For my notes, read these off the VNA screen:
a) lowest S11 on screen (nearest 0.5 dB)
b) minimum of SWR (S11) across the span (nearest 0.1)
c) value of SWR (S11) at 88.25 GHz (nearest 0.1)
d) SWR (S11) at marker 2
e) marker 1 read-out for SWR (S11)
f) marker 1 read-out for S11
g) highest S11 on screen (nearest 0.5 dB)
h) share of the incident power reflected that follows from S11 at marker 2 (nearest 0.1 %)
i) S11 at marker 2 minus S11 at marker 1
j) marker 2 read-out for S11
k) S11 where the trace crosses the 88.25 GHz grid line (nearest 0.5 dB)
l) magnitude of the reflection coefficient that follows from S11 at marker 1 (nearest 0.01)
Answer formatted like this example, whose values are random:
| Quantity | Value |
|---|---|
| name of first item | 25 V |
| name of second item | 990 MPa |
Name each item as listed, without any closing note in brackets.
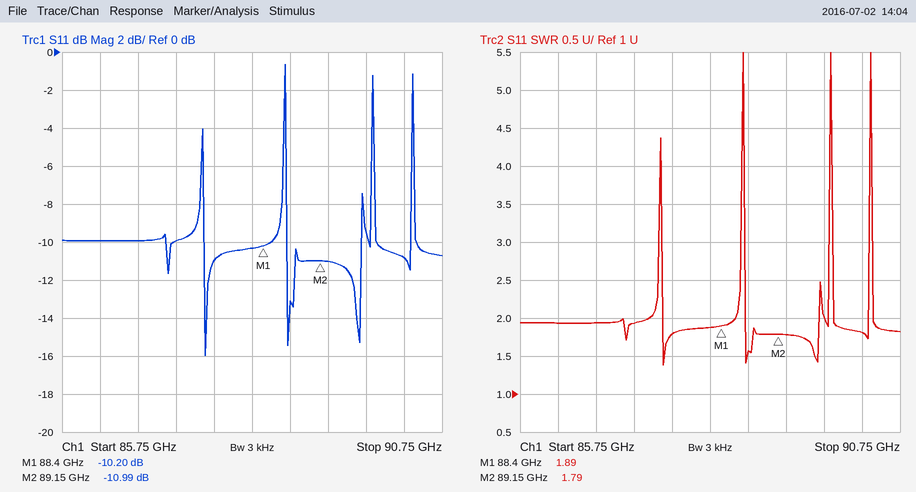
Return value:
| Quantity | Value |
|---|---|
| lowest S11 on screen | -16.0 dB |
| minimum of SWR (S11) across the span | 1.4 |
| value of SWR (S11) at 88.25 GHz | 1.9 |
| SWR (S11) at marker 2 | 1.79 |
| marker 1 read-out for SWR | 1.89 |
| marker 1 read-out for S11 | -10.20 dB |
| highest S11 on screen | -0.5 dB |
| share of the incident power reflected that follows from S11 at marker 2 | 8.0 % |
| S11 at marker 2 minus S11 at marker 1 | -0.79 dB |
| marker 2 read-out for S11 | -10.99 dB |
| S11 where the trace crosses the 88.25 GHz grid line | -10.5 dB |
| magnitude of the reflection coefficient that follows from S11 at marker 1 | 0.31 |
